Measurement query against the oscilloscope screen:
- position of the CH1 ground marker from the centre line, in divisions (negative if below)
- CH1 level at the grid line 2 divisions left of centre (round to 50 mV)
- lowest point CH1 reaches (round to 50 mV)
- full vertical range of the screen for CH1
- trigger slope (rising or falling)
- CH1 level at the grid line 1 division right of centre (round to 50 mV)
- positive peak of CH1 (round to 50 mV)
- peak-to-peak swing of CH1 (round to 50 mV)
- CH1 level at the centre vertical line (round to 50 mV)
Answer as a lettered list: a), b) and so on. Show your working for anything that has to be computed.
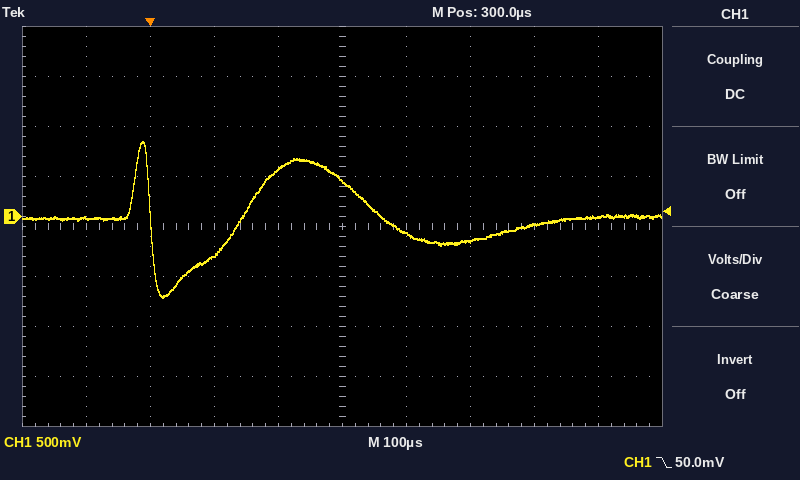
a) +0.2 div
b) -400 mV
c) -800 mV
d) 4 V
e) falling
f) -150 mV
g) 750 mV
h) 750 mV − (-800 mV) = 1.55 V
i) 350 mV
